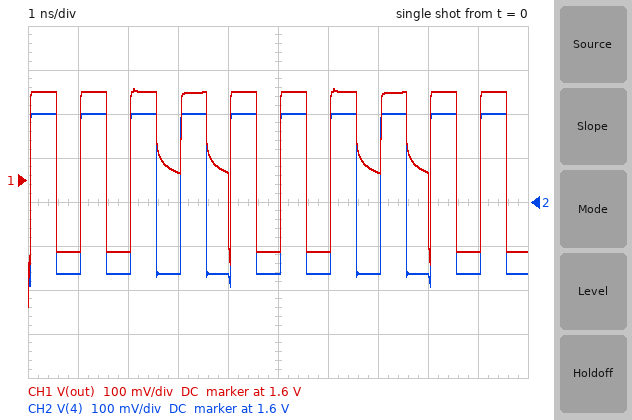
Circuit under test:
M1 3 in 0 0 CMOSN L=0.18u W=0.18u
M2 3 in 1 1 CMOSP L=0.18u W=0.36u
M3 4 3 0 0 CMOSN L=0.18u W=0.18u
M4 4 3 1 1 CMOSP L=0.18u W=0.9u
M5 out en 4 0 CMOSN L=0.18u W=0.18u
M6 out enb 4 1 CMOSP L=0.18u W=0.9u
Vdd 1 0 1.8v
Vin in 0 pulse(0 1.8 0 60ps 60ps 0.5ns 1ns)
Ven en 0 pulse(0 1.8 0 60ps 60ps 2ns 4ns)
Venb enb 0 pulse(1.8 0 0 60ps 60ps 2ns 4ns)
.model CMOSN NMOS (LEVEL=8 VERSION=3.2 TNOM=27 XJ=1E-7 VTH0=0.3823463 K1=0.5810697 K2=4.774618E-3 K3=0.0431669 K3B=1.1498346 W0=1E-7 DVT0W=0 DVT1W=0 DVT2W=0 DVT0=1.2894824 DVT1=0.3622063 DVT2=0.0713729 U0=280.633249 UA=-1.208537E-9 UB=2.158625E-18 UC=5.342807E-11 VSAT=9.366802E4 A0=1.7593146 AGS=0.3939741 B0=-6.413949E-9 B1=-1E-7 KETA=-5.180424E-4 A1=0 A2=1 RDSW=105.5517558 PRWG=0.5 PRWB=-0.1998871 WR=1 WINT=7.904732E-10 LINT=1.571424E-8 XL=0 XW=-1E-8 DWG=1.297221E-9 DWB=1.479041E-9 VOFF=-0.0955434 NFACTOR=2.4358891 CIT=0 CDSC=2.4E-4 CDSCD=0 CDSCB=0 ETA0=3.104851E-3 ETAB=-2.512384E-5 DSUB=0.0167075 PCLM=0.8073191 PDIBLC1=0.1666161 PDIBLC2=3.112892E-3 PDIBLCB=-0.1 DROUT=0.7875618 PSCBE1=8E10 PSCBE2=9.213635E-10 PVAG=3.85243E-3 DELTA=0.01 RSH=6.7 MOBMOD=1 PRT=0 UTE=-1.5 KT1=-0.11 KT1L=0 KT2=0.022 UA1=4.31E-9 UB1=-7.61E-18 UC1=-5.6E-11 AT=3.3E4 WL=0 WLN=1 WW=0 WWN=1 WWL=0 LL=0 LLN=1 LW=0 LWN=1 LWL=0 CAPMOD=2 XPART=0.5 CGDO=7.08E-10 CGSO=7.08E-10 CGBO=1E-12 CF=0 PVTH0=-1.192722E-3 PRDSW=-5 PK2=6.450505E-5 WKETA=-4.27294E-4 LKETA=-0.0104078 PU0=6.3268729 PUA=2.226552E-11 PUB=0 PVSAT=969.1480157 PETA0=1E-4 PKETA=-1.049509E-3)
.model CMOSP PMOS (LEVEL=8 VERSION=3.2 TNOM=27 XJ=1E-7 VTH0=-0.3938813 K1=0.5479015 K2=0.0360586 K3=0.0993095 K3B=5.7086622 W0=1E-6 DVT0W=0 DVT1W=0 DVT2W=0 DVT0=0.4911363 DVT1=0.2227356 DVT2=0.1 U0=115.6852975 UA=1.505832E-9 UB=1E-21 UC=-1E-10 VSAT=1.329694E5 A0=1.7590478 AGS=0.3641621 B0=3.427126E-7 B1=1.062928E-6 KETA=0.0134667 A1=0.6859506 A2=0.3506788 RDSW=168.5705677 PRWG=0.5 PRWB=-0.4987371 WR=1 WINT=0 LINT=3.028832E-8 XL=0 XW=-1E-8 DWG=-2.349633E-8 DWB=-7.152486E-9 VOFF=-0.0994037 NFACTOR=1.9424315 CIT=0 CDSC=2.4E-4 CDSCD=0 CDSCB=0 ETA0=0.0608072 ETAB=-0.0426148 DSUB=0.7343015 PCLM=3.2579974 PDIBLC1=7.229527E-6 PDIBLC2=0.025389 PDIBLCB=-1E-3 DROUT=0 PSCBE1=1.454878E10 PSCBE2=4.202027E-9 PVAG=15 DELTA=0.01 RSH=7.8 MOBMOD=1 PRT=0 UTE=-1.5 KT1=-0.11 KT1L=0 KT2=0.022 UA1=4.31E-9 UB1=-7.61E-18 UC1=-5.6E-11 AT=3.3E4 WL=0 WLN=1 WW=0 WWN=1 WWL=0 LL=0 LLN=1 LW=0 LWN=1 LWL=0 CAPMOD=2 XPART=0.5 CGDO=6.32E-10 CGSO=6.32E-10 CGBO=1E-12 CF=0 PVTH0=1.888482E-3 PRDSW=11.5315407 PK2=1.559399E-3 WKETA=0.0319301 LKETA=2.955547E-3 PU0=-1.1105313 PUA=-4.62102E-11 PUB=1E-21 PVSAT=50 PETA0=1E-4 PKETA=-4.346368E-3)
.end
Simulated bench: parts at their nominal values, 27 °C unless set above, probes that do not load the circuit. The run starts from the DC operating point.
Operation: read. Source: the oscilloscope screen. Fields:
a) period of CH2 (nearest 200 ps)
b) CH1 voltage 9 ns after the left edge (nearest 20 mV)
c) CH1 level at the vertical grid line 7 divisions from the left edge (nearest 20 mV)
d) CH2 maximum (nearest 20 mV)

1.0 ns
1.44 V
1.62 V
1.80 V
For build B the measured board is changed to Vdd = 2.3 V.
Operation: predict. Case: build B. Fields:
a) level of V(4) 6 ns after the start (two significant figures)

1.8 V
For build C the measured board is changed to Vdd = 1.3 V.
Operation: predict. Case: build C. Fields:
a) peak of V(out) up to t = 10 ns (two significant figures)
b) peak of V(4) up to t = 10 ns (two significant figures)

1.4 V
1.3 V
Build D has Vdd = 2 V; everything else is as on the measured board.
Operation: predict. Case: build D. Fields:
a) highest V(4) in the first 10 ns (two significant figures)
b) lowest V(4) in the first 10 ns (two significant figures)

1.7 V
1.6 V
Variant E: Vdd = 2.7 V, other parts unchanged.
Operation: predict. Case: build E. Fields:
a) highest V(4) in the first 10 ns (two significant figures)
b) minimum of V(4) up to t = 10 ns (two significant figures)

2.2 V
2.1 V
